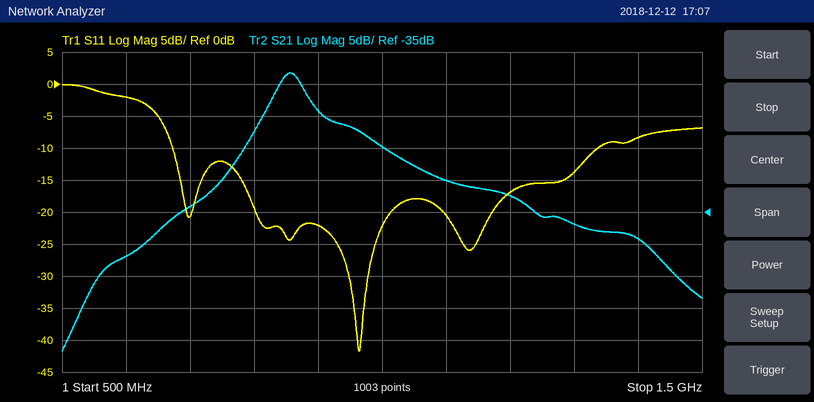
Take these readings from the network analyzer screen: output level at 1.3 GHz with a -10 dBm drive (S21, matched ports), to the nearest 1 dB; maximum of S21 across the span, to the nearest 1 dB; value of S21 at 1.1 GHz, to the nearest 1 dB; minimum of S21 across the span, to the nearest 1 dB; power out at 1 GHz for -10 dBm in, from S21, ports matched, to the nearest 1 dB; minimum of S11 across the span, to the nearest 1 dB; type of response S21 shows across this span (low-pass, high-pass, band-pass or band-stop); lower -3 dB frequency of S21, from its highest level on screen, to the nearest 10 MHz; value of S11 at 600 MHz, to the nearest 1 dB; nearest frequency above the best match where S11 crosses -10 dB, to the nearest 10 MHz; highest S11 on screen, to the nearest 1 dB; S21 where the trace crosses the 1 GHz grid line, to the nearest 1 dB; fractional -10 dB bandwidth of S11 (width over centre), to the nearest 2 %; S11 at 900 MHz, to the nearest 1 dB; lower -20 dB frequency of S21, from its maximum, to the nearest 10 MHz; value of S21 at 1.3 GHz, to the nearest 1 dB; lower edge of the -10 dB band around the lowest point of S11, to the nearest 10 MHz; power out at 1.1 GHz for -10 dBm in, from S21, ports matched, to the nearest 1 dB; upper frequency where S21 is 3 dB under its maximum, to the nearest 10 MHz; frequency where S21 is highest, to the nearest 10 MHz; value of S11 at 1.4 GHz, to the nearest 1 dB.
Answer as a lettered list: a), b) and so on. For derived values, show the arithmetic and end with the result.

a) -10 dBm + (-37 dB) = -47 dBm
b) -13 dB
c) -30 dB
d) -57 dB
e) -10 dBm + (-25 dB) = -35 dBm
f) -42 dB
g) band-pass
h) 830 MHz
i) -2 dB
j) 1.34 GHz
k) 0 dB
l) -25 dB
m) 670 MHz / 1.005 GHz ≈ 66.7 %, so 66 % to the nearest 2 %
n) -22 dB
o) 710 MHz
p) -37 dB
q) 670 MHz
r) -10 dBm + (-30 dB) = -40 dBm
s) 880 MHz
t) 860 MHz
u) -8 dB
